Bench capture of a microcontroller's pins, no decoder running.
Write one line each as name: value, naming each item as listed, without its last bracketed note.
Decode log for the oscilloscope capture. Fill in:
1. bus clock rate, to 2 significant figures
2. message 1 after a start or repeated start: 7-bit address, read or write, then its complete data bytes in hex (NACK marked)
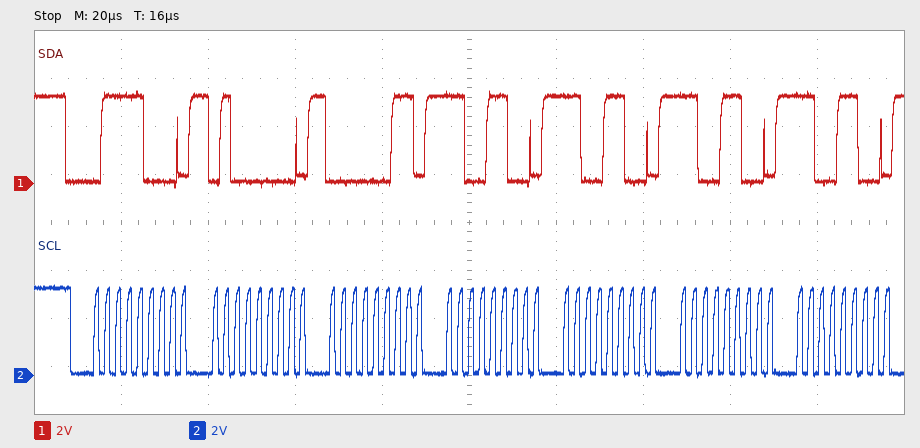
bus clock rate, to 2 significant figures: 400 kHz
message 1 after a start or repeated start: 7-bit address, read or write, then its complete data bytes in hex: 0x3C write: 40 03 CC CC CC CC
